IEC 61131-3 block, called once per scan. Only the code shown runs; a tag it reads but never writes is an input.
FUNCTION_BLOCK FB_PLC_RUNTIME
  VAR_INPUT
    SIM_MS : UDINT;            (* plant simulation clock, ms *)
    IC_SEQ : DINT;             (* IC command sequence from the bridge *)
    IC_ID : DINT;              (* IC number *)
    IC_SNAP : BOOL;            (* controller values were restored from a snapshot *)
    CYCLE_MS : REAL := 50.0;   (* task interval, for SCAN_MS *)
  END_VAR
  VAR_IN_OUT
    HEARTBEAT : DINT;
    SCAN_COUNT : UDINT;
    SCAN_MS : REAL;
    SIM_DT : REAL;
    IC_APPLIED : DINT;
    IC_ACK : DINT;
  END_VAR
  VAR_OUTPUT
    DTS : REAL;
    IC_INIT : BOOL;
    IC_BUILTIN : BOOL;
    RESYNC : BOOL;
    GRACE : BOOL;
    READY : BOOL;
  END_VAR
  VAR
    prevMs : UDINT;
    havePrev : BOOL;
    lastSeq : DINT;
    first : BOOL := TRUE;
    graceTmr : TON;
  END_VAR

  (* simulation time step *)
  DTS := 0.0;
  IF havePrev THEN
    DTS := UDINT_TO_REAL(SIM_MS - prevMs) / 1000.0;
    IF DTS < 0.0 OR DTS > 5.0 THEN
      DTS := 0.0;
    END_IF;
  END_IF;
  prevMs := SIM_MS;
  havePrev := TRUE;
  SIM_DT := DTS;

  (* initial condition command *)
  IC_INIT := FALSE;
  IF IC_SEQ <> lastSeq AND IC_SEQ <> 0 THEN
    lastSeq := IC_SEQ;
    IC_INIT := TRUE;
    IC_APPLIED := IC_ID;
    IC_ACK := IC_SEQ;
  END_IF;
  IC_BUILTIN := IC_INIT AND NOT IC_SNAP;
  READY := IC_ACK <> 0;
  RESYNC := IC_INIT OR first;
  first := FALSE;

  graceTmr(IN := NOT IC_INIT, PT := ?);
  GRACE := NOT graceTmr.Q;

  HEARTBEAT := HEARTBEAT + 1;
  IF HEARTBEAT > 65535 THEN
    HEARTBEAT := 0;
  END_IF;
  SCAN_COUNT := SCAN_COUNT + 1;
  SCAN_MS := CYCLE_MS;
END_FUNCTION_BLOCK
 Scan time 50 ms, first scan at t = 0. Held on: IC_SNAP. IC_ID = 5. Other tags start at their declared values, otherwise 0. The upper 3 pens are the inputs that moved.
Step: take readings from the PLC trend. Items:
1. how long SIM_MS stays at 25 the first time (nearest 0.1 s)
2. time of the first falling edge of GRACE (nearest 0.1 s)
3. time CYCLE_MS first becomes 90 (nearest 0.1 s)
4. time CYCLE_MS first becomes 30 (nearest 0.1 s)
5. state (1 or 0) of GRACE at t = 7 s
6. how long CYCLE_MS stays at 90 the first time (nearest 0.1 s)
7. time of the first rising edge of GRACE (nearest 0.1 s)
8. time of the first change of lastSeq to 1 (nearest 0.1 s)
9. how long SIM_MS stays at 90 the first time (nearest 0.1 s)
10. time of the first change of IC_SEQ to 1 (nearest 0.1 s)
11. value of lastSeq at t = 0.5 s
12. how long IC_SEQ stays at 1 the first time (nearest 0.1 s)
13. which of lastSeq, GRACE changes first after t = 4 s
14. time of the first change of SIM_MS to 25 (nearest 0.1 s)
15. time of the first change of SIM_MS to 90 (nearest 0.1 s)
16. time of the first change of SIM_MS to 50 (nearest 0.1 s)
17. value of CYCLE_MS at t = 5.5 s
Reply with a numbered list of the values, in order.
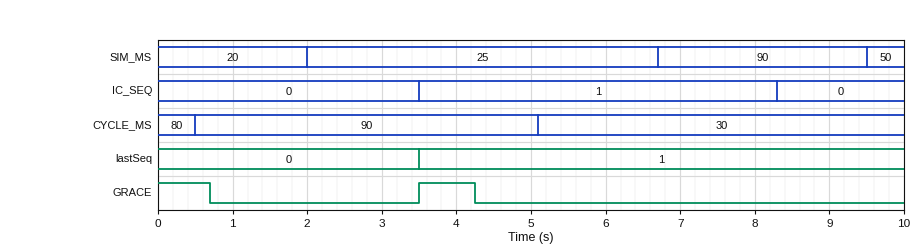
1. 4.7 s
2. 0.7 s
3. 0.5 s
4. 5.1 s
5. 0
6. 4.6 s
7. 3.5 s
8. 3.5 s
9. 2.8 s
10. 3.5 s
11. 0
12. 4.8 s
13. GRACE
14. 2.0 s
15. 6.7 s
16. 9.5 s
17. 30
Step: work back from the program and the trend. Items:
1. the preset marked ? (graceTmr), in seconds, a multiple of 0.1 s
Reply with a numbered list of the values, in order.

1. 0.7 s
